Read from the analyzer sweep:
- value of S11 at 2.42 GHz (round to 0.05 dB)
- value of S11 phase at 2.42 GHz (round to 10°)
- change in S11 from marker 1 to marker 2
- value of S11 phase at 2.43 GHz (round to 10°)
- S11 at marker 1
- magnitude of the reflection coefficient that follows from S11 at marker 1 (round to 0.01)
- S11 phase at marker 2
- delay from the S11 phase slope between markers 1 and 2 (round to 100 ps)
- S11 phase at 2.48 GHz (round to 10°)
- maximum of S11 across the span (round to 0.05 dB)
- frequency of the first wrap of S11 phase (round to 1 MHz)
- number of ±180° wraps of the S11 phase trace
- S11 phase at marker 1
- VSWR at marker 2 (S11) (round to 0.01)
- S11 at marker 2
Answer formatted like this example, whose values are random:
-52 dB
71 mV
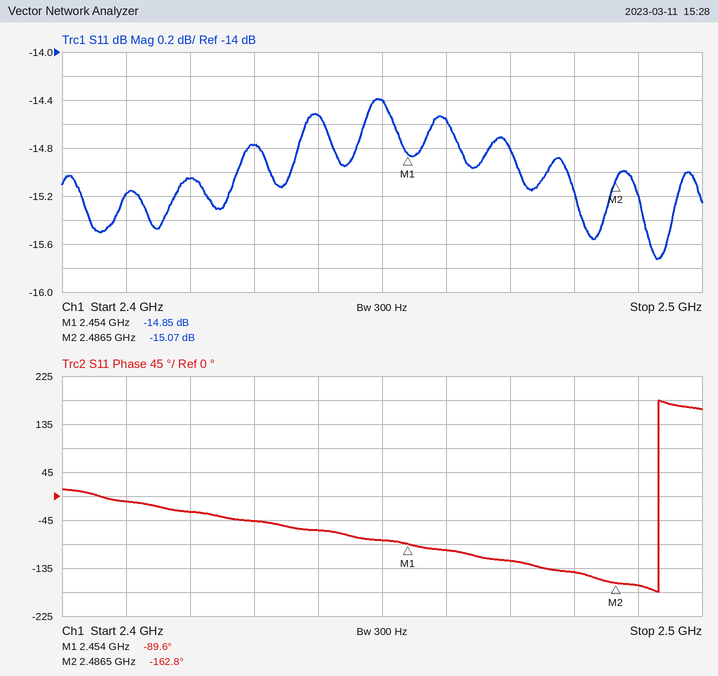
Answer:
-15.05 dB
-30°
-0.22 dB
-50°
-14.85 dB
0.18
-162.8°
6.3 ns
-140°
-14.40 dB
2.493 GHz
1
-89.6°
1.43
-15.07 dB
